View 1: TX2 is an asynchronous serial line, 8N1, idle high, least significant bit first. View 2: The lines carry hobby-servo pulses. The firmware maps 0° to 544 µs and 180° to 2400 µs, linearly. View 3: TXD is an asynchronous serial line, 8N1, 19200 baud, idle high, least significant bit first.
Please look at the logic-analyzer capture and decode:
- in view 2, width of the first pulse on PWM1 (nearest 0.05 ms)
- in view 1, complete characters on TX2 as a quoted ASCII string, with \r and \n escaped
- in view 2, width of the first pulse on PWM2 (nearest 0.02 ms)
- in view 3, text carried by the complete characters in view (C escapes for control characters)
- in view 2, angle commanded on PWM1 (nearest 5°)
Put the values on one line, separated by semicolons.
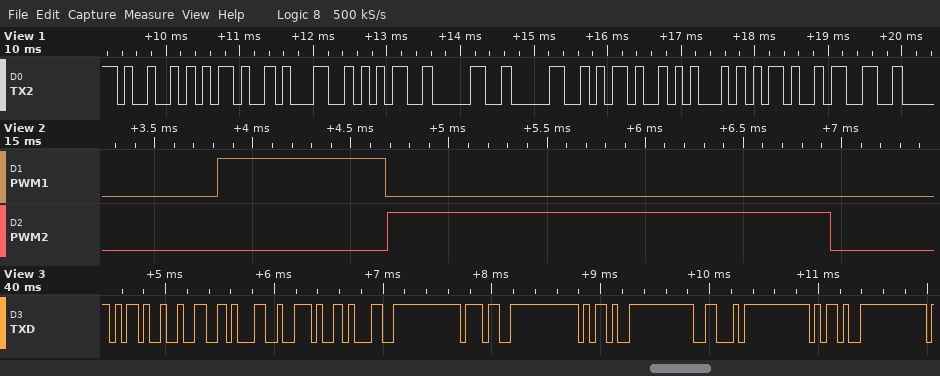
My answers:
0.85 ms; "I-1500-E-3"; 2.26 ms; "-21.17-F-"; 30°
